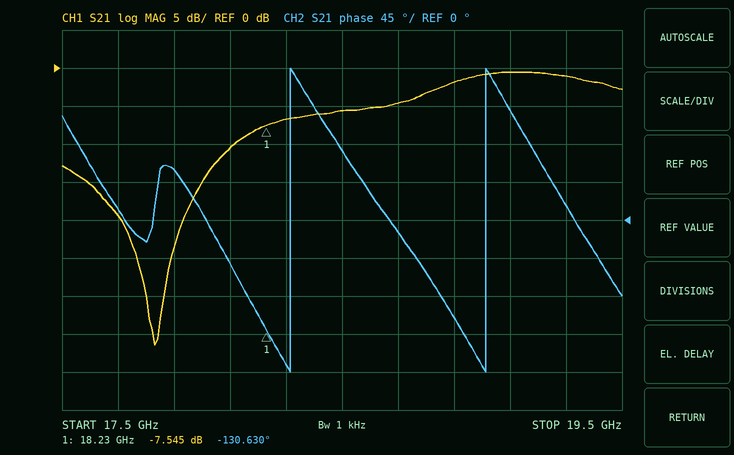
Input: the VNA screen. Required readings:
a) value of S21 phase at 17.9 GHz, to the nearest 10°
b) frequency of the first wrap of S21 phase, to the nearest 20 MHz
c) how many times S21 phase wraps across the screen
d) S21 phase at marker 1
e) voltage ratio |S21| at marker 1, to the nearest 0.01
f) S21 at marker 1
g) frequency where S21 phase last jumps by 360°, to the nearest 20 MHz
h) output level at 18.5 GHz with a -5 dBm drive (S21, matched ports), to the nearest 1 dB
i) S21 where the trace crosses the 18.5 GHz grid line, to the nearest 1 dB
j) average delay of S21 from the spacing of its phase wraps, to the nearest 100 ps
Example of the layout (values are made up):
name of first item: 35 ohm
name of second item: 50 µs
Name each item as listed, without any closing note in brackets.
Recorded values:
value of S21 phase at 17.9 GHz, to the nearest 10°: 60°
frequency of the first wrap of S21 phase, to the nearest 20 MHz: 18.32 GHz
how many times S21 phase wraps across the screen: 2
S21 phase at marker 1: -130.630°
voltage ratio |S21| at marker 1, to the nearest 0.01: 0.42
S21 at marker 1: -7.545 dB
frequency where S21 phase last jumps by 360°, to the nearest 20 MHz: 19.02 GHz
output level at 18.5 GHz with a -5 dBm drive (S21, matched ports), to the nearest 1 dB: -11 dBm
S21 where the trace crosses the 18.5 GHz grid line, to the nearest 1 dB: -6 dB
average delay of S21 from the spacing of its phase wraps, to the nearest 100 ps: 1.4 ns
